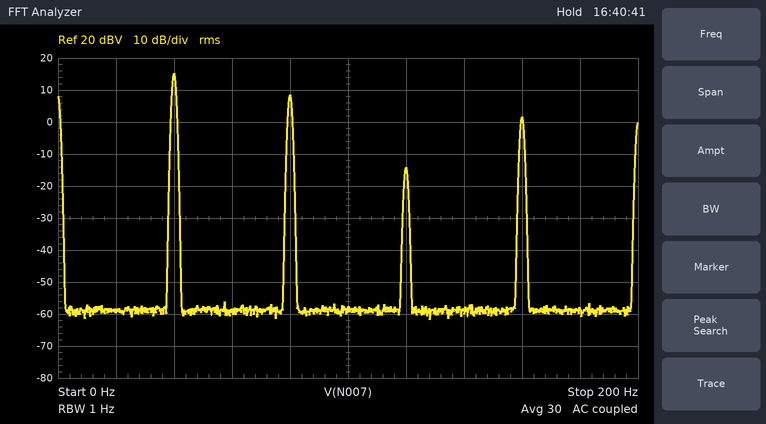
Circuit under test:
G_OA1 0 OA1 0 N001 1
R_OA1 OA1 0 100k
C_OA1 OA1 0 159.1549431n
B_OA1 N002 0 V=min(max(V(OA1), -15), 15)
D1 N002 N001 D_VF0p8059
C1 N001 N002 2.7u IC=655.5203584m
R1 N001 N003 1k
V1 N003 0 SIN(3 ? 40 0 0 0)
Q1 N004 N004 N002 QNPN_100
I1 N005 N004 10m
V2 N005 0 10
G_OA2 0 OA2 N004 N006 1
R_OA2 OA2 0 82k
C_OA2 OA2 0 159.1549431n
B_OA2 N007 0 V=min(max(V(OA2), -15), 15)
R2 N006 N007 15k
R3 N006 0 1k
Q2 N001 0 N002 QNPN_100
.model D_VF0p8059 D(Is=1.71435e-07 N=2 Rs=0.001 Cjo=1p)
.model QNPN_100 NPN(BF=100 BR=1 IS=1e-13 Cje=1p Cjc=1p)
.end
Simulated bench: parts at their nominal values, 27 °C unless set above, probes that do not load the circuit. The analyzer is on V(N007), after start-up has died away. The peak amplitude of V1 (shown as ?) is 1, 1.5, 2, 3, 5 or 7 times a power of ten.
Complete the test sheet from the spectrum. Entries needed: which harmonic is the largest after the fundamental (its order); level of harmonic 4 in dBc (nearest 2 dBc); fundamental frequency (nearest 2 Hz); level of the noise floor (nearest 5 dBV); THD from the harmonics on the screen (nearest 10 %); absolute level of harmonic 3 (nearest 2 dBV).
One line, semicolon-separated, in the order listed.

2; -14 dBc; 40 Hz; -60 dBV; 50 %; -14 dBV
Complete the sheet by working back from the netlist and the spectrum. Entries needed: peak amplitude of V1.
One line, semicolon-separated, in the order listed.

5 V
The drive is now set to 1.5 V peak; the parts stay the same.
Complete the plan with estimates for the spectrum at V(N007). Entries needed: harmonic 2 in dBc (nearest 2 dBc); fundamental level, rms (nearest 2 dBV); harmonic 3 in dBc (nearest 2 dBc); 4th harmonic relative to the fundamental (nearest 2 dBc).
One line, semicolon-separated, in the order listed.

-18 dBc; -16 dBV; -32 dBc; -46 dBc
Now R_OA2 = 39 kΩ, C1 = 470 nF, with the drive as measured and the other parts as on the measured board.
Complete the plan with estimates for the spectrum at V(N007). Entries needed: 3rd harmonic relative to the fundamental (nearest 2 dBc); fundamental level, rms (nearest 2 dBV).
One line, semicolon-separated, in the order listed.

-34 dBc; 16 dBV
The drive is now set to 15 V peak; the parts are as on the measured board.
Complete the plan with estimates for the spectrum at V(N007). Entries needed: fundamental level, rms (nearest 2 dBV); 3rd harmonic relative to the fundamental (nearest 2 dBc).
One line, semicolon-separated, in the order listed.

16 dBV; -10 dBc
